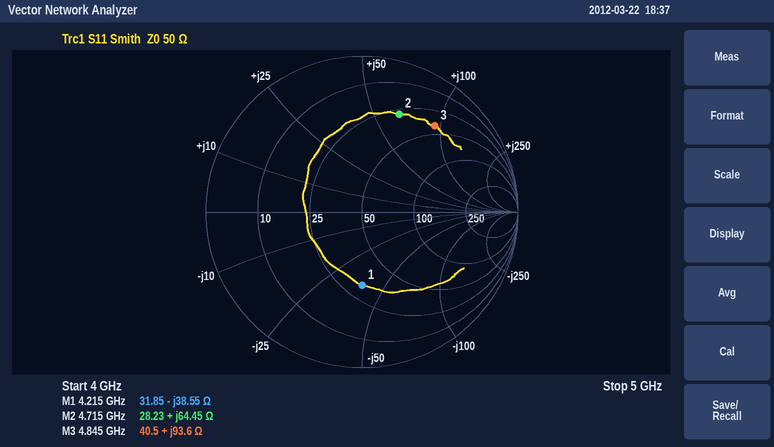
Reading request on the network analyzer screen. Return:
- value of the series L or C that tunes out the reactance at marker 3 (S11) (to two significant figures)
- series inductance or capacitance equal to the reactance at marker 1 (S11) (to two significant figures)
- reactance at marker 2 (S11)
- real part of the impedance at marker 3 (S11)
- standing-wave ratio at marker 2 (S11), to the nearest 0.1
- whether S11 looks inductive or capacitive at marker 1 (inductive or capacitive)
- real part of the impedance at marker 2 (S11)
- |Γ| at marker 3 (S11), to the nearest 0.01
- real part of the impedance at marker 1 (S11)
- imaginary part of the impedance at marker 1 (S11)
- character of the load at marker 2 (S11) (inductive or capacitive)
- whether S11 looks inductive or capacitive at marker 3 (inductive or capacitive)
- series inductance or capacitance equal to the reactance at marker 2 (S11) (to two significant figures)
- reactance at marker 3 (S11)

350 fF
980 fF
+64.45 Ω
40.5 Ω
5.1
capacitive
28.23 Ω
0.72
31.85 Ω
-38.55 Ω
inductive
inductive
2.2 nH
+93.6 Ω
